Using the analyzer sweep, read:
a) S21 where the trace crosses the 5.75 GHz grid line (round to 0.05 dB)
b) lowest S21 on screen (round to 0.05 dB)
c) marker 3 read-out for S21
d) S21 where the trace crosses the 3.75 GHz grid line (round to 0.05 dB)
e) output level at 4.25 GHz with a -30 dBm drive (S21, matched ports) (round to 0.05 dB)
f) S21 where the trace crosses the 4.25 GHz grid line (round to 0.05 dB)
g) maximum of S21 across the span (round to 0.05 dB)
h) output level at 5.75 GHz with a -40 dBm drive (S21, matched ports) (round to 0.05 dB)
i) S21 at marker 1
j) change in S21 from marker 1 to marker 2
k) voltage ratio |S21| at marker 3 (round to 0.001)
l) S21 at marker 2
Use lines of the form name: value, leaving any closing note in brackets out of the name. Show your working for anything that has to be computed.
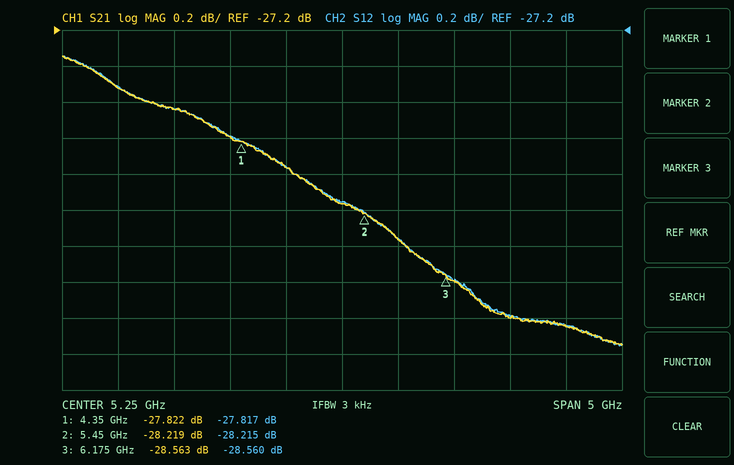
S21 where the trace crosses the 5.75 GHz grid line: -28.35 dB
lowest S21 on screen: -28.95 dB
marker 3 read-out for S21: -28.563 dB
S21 where the trace crosses the 3.75 GHz grid line: -27.65 dB
output level at 4.25 GHz with a -30 dBm drive (S21, matched ports): -30 dBm + (-27.80 dB) = -57.80 dBm
S21 where the trace crosses the 4.25 GHz grid line: -27.80 dB
maximum of S21 across the span: -27.35 dB
output level at 5.75 GHz with a -40 dBm drive (S21, matched ports): -40 dBm + (-28.35 dB) = -68.35 dBm
S21 at marker 1: -27.822 dB
change in S21 from marker 1 to marker 2: -28.219 − (-27.822) = -0.397 dB
voltage ratio |S21| at marker 3: 10^(-28.563/20) ≈ 0.037
S21 at marker 2: -28.219 dB
